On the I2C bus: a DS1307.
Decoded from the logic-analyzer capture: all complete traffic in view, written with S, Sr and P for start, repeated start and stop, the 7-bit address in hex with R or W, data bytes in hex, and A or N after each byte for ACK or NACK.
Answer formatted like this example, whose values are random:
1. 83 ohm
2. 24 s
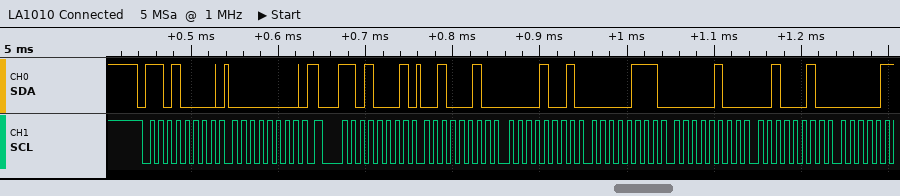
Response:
1. S 68W A 00 A Sr 68R A 22 A 09 A 07 A 04 A 22 A
